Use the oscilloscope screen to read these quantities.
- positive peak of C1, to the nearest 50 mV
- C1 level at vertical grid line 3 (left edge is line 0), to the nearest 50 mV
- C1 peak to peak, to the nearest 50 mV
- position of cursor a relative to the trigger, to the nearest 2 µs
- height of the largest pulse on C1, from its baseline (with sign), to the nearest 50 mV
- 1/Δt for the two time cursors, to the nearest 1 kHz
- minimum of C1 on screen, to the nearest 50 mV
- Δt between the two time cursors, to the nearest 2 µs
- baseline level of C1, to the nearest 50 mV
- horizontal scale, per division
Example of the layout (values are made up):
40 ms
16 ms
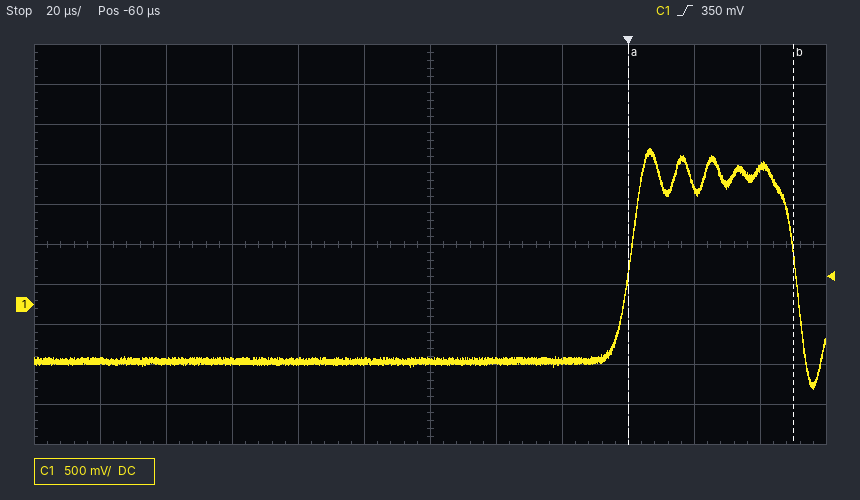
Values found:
1.95 V
-700 mV
3.00 V
0 µs
+2.65 V
20 kHz
-1.05 V
50 µs
-700 mV
20 µs
